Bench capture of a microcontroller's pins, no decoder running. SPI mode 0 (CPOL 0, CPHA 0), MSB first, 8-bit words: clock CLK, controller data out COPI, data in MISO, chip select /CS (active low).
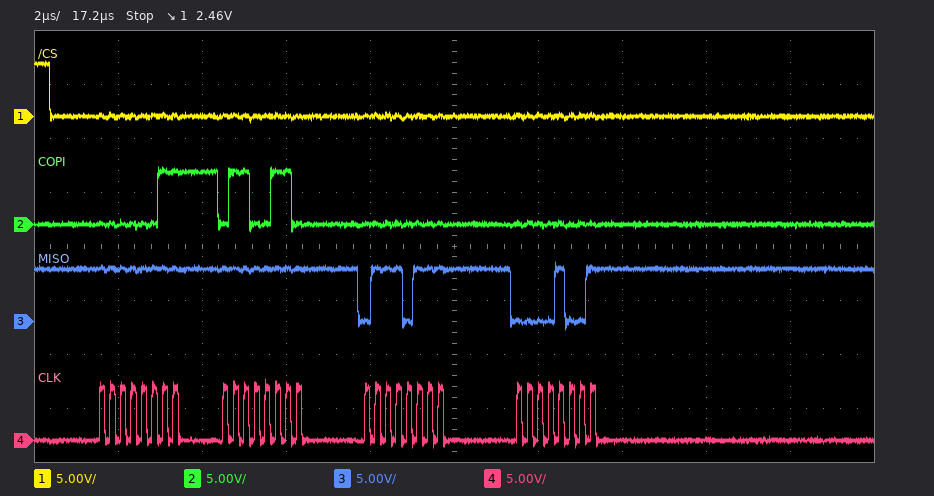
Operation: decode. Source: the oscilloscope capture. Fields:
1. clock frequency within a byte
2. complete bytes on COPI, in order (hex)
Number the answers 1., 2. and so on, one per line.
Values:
1. 4 MHz
2. 0x03 0x66 0x00 0x00
